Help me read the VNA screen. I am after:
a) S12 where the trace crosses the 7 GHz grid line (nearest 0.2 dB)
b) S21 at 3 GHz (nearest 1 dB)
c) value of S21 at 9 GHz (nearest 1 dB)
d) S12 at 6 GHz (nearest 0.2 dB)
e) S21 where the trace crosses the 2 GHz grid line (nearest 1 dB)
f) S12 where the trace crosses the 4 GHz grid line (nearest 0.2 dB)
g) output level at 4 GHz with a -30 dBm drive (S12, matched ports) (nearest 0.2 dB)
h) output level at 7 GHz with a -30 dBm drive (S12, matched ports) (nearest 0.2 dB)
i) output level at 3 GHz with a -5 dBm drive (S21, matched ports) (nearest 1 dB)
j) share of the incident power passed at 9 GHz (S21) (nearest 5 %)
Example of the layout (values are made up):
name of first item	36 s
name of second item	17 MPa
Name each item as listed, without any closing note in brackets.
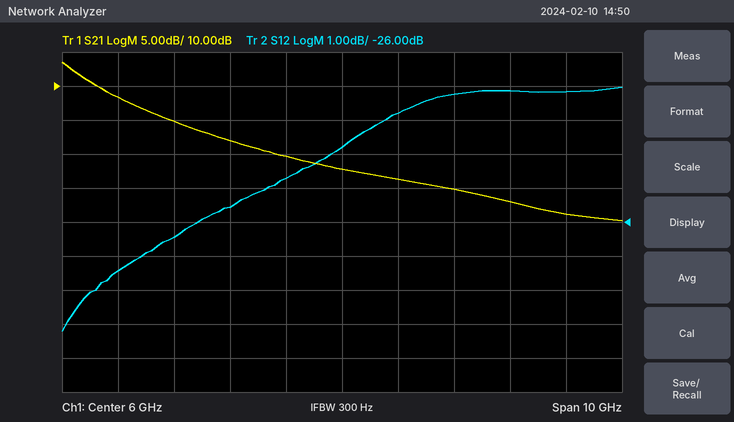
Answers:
S12 where the trace crosses the 7 GHz grid line	-22.8 dB
S21 at 3 GHz	5 dB
value of S21 at 9 GHz	-7 dB
S12 at 6 GHz	-23.8 dB
S21 where the trace crosses the 2 GHz grid line	8 dB
S12 where the trace crosses the 4 GHz grid line	-25.6 dB
output level at 4 GHz with a -30 dBm drive (S12, matched ports)	-55.6 dBm
output level at 7 GHz with a -30 dBm drive (S12, matched ports)	-52.8 dBm
output level at 3 GHz with a -5 dBm drive (S21, matched ports)	0 dBm
share of the incident power passed at 9 GHz (S21)	20 %
